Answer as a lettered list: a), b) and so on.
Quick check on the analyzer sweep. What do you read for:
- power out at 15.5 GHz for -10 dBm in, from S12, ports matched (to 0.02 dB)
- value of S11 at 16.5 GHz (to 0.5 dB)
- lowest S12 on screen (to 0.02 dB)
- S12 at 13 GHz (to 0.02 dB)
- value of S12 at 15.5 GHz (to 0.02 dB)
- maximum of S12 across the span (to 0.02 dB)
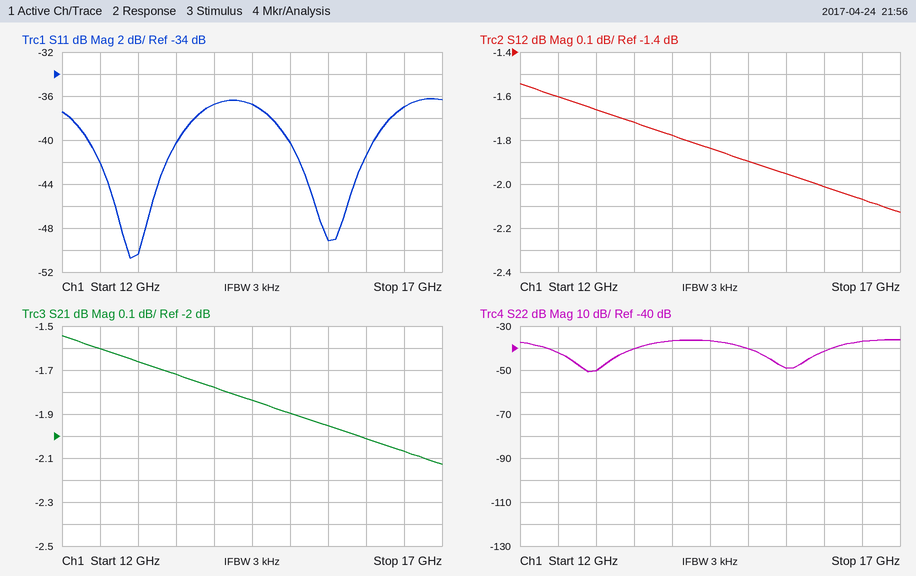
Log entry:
a) -11.96 dBm
b) -37.0 dB
c) -2.12 dB
d) -1.66 dB
e) -1.96 dB
f) -1.54 dB
